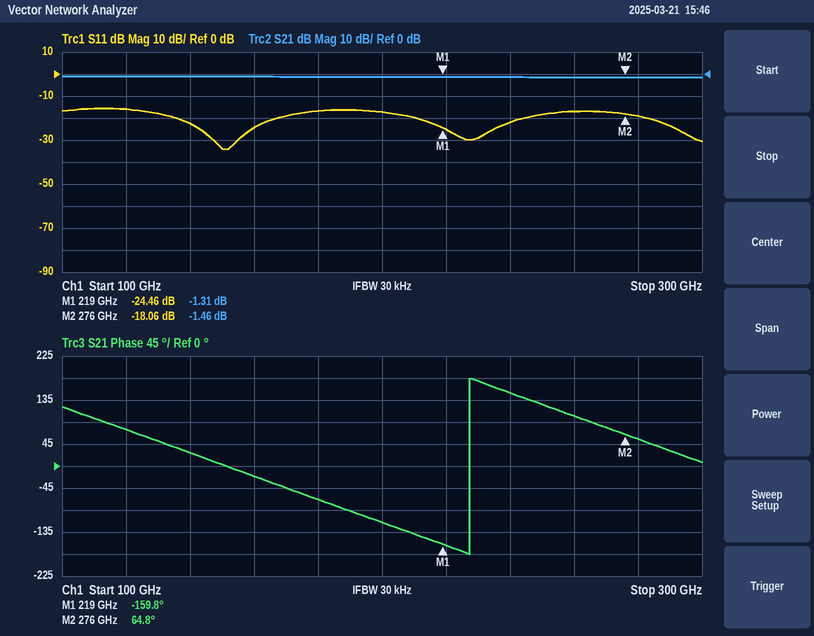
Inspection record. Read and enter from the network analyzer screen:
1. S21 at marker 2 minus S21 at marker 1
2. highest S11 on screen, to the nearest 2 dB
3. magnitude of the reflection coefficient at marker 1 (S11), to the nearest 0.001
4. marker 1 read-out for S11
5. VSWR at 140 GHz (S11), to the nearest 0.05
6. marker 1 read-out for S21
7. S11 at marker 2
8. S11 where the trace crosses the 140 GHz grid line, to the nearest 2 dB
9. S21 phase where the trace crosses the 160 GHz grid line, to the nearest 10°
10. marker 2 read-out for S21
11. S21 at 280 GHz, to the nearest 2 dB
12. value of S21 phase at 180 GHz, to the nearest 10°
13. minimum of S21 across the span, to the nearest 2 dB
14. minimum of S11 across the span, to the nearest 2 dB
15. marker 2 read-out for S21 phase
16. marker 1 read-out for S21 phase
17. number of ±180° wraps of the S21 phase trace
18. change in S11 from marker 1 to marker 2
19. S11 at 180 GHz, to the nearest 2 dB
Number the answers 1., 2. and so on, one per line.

1. -0.15 dB
2. -16 dB
3. 0.060
4. -24.46 dB
5. 1.15
6. -1.31 dB
7. -18.06 dB
8. -22 dB
9. -20°
10. -1.46 dB
11. -2 dB
12. -70°
13. -2 dB
14. -34 dB
15. 64.8°
16. -159.8°
17. 1
18. 6.40 dB
19. -16 dB
